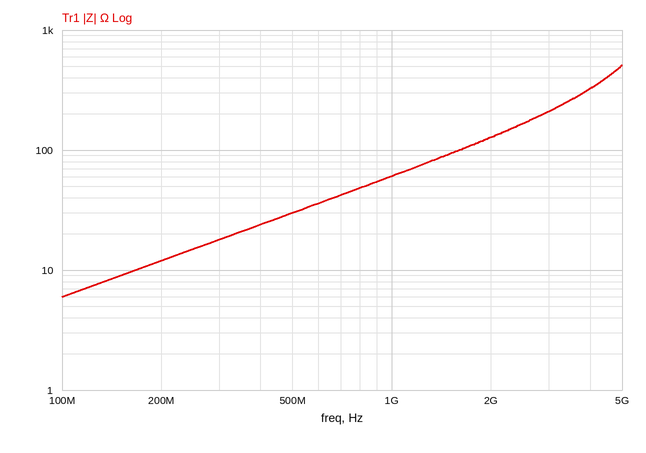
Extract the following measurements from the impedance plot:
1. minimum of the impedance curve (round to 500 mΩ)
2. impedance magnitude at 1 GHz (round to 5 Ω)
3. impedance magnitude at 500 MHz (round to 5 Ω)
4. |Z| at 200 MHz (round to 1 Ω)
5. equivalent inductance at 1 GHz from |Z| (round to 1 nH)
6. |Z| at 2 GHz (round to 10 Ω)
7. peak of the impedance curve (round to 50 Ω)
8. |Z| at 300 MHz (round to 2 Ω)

6.0 Ω
60 Ω
30 Ω
12 Ω
10 nH
130 Ω
500 Ω
18 Ω
